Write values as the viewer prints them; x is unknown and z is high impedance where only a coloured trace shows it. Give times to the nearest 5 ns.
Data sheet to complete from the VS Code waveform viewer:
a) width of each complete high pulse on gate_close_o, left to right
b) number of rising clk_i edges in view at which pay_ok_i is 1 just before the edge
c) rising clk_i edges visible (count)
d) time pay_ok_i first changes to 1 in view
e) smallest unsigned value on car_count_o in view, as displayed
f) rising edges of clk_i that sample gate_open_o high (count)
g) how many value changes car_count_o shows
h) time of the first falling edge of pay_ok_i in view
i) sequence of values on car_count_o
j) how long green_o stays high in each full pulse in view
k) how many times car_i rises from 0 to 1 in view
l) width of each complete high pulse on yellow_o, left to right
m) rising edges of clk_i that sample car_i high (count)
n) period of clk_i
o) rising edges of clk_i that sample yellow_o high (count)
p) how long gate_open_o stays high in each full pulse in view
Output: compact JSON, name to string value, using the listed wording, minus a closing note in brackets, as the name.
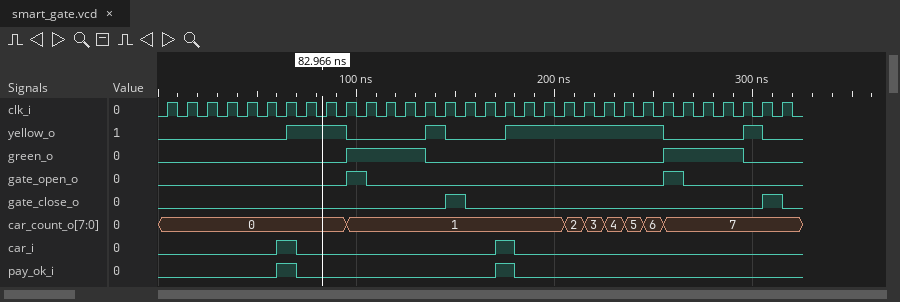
{"width of each complete high pulse on gate_close_o, left to right": "10 ns, 10 ns", "number of rising clk_i edges in view at which pay_ok_i is 1 just before the edge": "2", "rising clk_i edges visible": "32", "time pay_ok_i first changes to 1 in view": "60 ns", "smallest unsigned value on car_count_o in view, as displayed": "0", "rising edges of clk_i that sample gate_open_o high": "2", "how many value changes car_count_o shows": "7", "time of the first falling edge of pay_ok_i in view": "70 ns", "sequence of values on car_count_o": "0, 1, 2, 3, 4, 5, 6, 7", "how long green_o stays high in each full pulse in view": "40 ns, 40 ns", "how many times car_i rises from 0 to 1 in view": "2", "width of each complete high pulse on yellow_o, left to right": "30 ns, 10 ns, 80 ns, 10 ns", "rising edges of clk_i that sample car_i high": "2", "period of clk_i": "10 ns", "rising edges of clk_i that sample yellow_o high": "13", "how long gate_open_o stays high in each full pulse in view": "10 ns, 10 ns"}
